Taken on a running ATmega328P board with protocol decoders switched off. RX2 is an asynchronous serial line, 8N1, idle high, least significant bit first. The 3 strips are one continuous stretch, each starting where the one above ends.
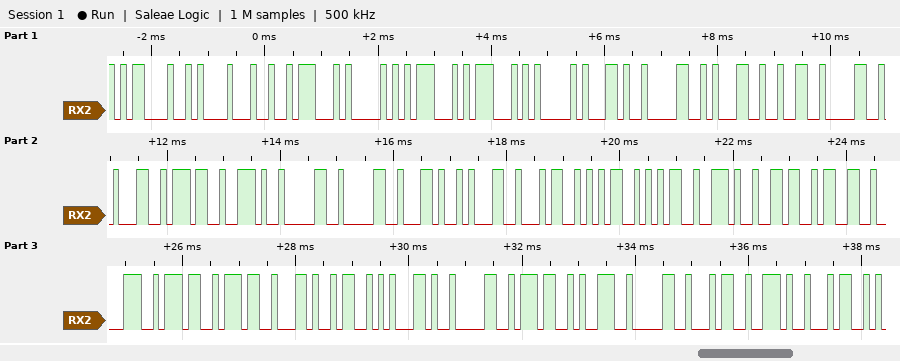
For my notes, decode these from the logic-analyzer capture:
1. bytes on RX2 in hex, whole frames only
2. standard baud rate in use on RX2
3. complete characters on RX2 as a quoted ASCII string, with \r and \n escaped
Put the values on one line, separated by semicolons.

0D 0A 24 47 50 47 47 41 2C 30 31 32 30 31 37 2E 30 30 2C 31 34 35 35 2E 36 33 38 37 37 2C 53 2C 30 37 39 30 34 2E 34; 9600 baud; "\r\n$GPGGA,012017.00,1455.63877,S,07904.4"
